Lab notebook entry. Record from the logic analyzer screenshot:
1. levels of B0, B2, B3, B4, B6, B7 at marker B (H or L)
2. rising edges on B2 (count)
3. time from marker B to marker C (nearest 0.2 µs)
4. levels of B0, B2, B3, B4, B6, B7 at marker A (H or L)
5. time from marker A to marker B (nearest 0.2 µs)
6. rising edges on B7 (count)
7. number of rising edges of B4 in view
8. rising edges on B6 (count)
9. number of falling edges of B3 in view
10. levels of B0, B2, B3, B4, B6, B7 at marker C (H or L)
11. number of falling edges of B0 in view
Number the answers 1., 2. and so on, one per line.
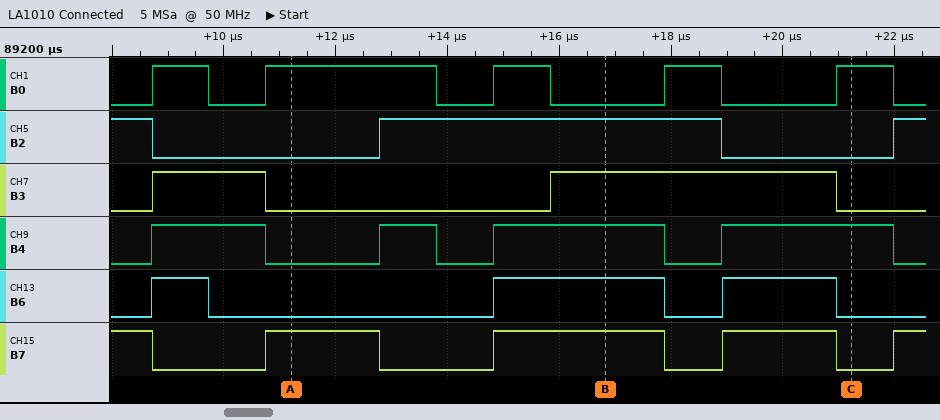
1. B0=L, B2=H, B3=H, B4=H, B6=H, B7=H
2. 2
3. 4.4 µs
4. B0=H, B2=L, B3=L, B4=L, B6=L, B7=H
5. 5.6 µs
6. 4
7. 4
8. 3
9. 2
10. B0=H, B2=L, B3=L, B4=H, B6=L, B7=L
11. 5
